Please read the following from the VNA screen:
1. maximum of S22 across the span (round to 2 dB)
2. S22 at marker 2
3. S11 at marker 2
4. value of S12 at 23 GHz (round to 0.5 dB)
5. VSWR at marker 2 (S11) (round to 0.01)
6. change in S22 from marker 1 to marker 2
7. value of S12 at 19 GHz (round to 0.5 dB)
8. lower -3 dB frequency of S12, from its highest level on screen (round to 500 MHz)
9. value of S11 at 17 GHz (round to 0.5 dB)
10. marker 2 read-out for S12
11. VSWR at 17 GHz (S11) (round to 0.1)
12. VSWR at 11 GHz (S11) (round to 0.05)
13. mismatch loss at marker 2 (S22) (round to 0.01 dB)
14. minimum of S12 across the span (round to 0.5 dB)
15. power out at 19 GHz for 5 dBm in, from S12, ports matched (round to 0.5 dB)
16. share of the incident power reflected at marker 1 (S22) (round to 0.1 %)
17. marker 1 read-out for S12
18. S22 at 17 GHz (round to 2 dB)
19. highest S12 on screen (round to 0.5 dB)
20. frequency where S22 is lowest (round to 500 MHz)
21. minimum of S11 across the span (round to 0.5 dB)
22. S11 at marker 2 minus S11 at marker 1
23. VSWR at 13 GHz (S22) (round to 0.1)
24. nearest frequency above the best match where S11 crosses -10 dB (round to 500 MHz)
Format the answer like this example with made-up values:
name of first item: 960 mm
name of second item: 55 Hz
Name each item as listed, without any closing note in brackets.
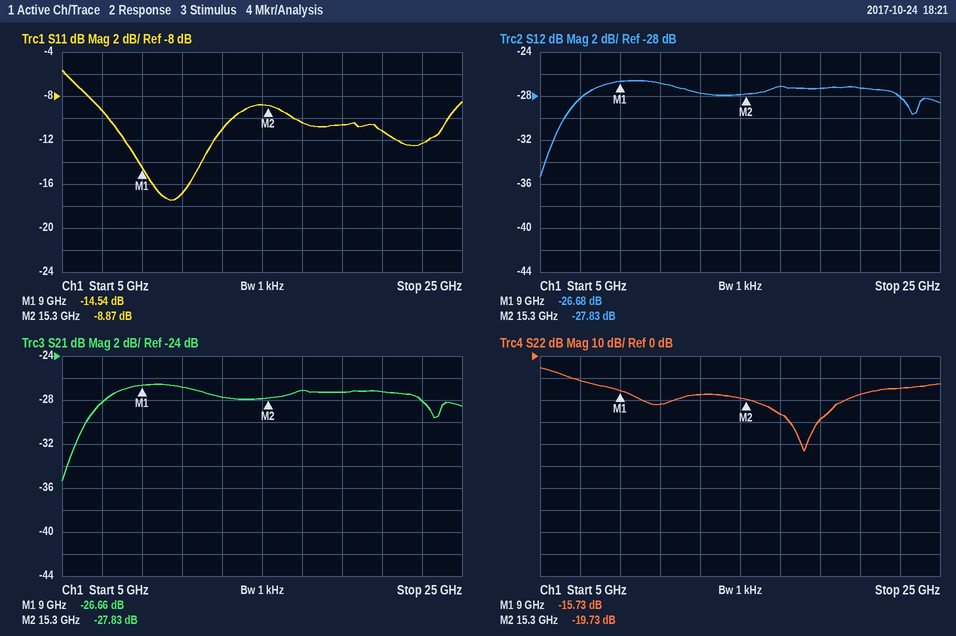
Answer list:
maximum of S22 across the span: -6 dB
S22 at marker 2: -19.73 dB
S11 at marker 2: -8.87 dB
value of S12 at 23 GHz: -28.0 dB
VSWR at marker 2 (S11): 2.13
change in S22 from marker 1 to marker 2: -4.00 dB
value of S12 at 19 GHz: -27.5 dB
lower -3 dB frequency of S12, from its highest level on screen: 6.5 GHz
value of S11 at 17 GHz: -10.5 dB
marker 2 read-out for S12: -27.83 dB
VSWR at 17 GHz (S11): 1.9
VSWR at 11 GHz (S11): 1.35
mismatch loss at marker 2 (S22): 0.05 dB
minimum of S12 across the span: -35.5 dB
power out at 19 GHz for 5 dBm in, from S12, ports matched: -22.5 dBm
share of the incident power reflected at marker 1 (S22): 2.7 %
marker 1 read-out for S12: -26.68 dB
S22 at 17 GHz: -26 dB
highest S12 on screen: -26.5 dB
frequency where S22 is lowest: 18.0 GHz
minimum of S11 across the span: -17.5 dB
S11 at marker 2 minus S11 at marker 1: 5.67 dB
VSWR at 13 GHz (S22): 1.3
nearest frequency above the best match where S11 crosses -10 dB: 13.5 GHz
